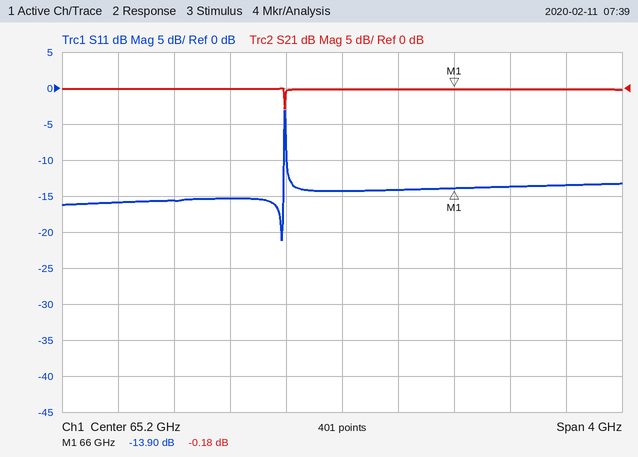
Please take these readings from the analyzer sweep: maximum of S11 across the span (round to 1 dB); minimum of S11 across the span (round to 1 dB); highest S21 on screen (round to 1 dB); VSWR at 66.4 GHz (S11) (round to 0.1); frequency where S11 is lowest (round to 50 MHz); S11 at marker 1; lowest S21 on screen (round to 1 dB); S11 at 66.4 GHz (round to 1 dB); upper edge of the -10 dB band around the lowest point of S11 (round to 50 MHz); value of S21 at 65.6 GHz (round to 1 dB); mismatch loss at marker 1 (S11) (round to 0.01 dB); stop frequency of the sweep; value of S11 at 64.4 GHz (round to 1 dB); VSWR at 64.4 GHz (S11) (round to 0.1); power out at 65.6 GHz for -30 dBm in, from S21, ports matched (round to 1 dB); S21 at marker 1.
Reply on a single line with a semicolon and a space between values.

-3 dB; -21 dB; 0 dB; 1.5; 64.75 GHz; -13.90 dB; -3 dB; -14 dB; 64.80 GHz; 0 dB; 0.18 dB; 67.2 GHz; -15 dB; 1.4; -30 dBm; -0.18 dB
